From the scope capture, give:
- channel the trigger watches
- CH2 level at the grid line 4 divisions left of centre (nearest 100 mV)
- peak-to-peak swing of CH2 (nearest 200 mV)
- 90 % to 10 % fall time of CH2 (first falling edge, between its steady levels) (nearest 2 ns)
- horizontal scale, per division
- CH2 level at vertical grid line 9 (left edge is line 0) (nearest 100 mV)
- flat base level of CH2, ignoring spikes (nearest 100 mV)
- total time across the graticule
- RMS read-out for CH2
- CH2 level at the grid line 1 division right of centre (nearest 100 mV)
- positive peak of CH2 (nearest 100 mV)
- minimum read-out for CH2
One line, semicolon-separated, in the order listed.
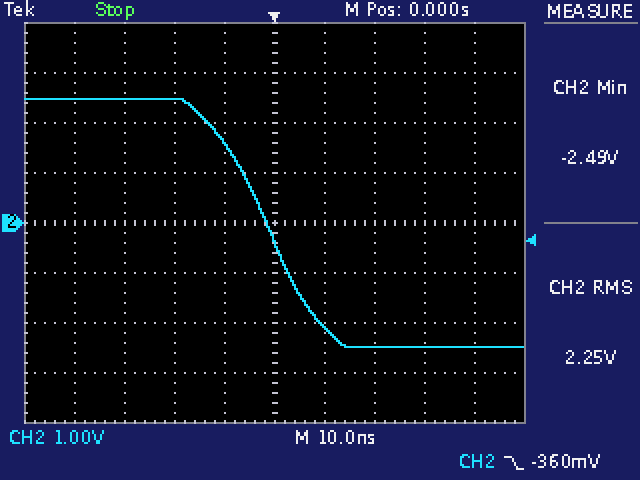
CH2; 2.5 V; 5.0 V; 22 ns; 10 ns; -2.5 V; -2.5 V; 100 ns; 2.25 V; -2.1 V; 2.5 V; -2.49 V
